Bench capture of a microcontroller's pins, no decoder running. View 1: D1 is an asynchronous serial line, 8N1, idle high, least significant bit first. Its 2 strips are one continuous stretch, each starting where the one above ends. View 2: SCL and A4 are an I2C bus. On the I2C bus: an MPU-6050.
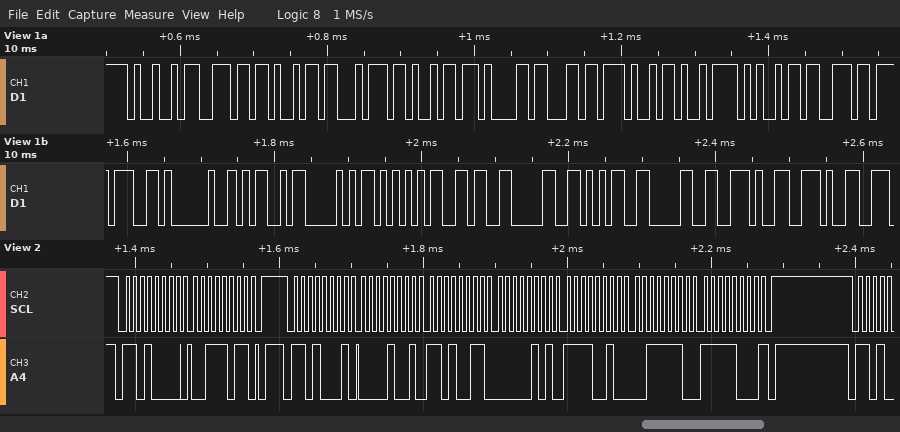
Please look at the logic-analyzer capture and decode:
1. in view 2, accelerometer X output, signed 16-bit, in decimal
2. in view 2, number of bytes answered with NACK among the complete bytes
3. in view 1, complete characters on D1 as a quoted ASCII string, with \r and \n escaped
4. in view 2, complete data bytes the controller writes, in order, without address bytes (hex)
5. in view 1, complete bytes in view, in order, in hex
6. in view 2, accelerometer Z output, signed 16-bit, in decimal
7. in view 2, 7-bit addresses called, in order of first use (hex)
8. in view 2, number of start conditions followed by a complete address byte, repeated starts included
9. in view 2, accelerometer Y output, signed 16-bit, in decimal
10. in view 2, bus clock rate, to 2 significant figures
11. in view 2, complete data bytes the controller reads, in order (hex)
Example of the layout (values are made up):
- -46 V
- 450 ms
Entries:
- 2515
- 1
- "Initializing MPU6050.."
- 3B
- 49 6E 69 74 69 61 6C 69 7A 69 6E 67 20 4D 50 55 36 30 35 30 2E 2E
- 16120
- 0x68
- 2
- 1522
- 100 kHz
- 09 D3 05 F2 3E F8
